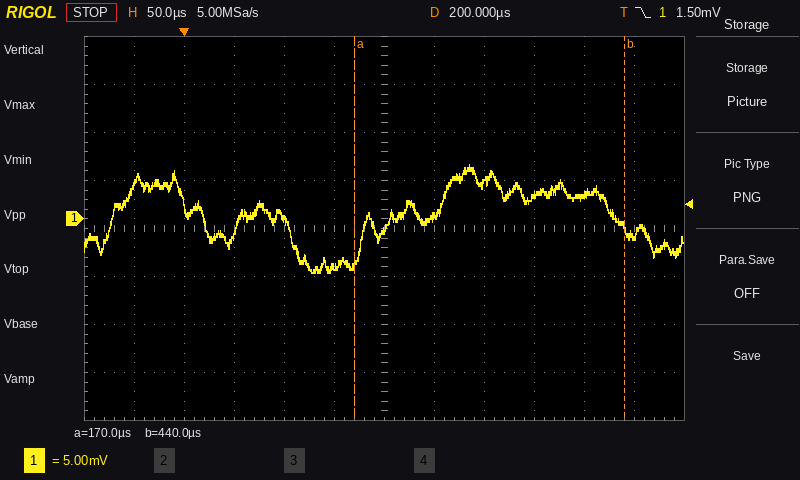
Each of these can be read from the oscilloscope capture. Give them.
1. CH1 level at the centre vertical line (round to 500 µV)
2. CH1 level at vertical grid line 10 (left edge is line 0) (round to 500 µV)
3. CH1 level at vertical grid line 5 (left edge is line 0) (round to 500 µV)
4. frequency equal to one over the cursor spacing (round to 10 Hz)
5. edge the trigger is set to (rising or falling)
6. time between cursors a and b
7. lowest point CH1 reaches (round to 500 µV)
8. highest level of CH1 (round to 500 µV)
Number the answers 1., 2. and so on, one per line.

1. -1.0 mV
2. 2.5 mV
3. -5.0 mV
4. 3.70 kHz
5. falling
6. 270 µs
7. -5.5 mV
8. 5.5 mV
